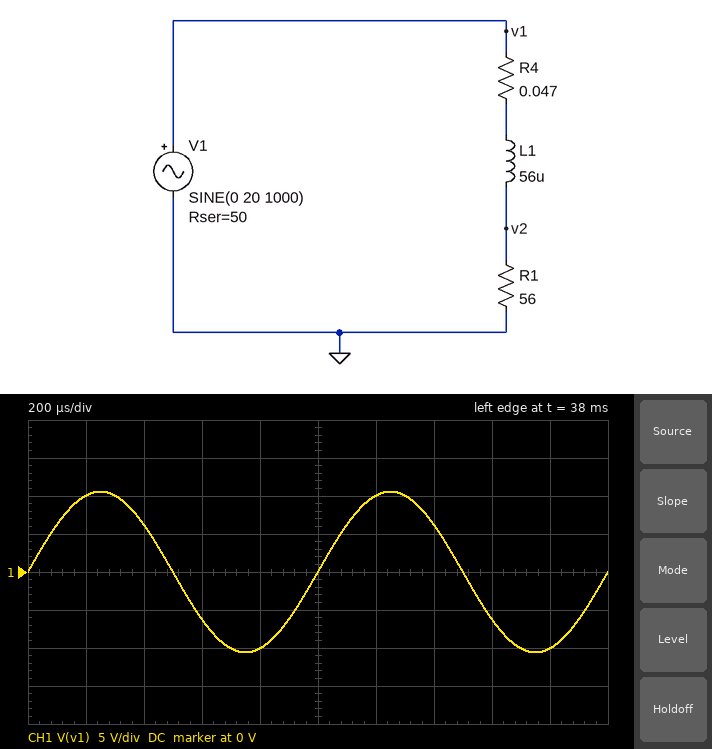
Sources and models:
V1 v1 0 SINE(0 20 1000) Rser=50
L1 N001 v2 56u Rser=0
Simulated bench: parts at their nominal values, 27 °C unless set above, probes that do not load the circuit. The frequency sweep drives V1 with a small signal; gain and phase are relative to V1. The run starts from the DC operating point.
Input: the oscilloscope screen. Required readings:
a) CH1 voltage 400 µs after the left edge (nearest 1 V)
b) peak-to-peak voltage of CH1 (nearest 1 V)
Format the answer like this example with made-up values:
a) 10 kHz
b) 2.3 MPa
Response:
a) 6 V
b) 21 V
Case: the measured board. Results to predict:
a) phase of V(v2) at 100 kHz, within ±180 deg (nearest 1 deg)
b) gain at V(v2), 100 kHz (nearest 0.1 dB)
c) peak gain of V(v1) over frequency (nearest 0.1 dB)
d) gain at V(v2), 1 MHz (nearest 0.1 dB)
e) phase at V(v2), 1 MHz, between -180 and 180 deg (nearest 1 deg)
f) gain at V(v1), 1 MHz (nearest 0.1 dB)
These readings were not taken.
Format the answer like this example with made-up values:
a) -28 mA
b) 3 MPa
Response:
a) -18 deg
b) -6.0 dB
c) 0 dB
d) -16.3 dB
e) -73 deg
f) -0.3 dB
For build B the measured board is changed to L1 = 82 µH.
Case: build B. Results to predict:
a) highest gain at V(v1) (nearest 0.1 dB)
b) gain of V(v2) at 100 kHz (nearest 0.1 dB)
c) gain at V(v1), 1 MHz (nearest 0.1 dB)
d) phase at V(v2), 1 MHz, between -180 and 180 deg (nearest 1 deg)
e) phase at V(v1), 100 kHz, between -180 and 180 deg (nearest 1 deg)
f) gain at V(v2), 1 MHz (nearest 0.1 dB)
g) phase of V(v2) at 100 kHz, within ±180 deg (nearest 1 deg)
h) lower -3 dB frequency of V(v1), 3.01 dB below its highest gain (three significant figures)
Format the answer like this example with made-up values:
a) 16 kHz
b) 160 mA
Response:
a) 0 dB
b) -6.5 dB
c) -0.1 dB
d) -78 deg
e) 17 deg
f) -19.5 dB
g) -26 deg
h) 137 kHz
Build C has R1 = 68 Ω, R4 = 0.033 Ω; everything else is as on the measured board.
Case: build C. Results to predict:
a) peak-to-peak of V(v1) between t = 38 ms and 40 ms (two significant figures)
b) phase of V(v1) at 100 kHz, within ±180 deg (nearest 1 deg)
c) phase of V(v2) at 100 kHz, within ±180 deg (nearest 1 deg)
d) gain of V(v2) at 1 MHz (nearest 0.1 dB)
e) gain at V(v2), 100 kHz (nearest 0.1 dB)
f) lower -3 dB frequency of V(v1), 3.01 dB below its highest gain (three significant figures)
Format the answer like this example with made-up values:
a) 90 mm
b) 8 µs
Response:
a) 23 V
b) 11 deg
c) -17 deg
d) -14.7 dB
e) -5.2 dB
f) 194 kHz
